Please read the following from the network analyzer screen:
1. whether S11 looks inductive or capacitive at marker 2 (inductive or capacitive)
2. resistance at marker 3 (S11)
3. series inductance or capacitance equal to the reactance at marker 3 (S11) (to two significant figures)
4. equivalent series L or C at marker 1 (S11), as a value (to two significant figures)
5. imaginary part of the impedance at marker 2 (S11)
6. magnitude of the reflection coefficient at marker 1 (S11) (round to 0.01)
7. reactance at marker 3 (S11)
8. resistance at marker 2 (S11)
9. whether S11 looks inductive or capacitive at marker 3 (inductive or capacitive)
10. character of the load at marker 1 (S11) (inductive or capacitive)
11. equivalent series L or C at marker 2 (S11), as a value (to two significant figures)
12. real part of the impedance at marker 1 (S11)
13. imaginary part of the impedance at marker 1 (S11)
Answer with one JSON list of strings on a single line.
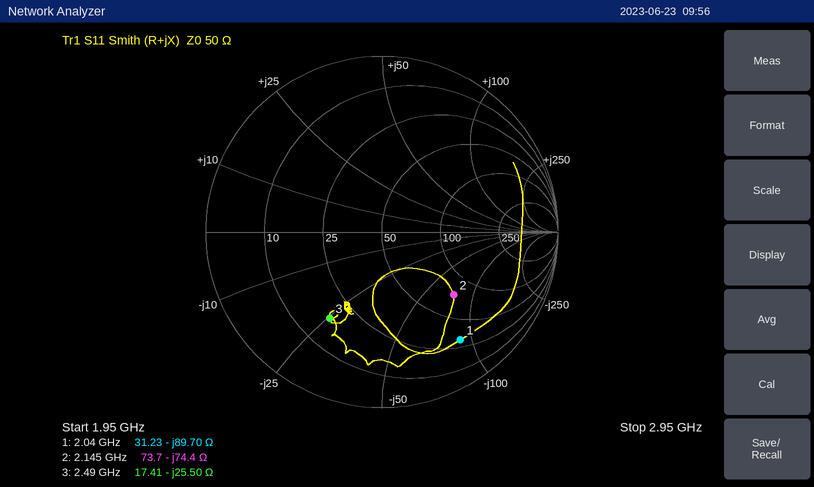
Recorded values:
["capacitive", "17.41 Ω", "2.5 pF", "870 fF", "-74.4 Ω", "0.76", "-25.50 Ω", "73.7 Ω", "capacitive", "capacitive", "1.00 pF", "31.23 Ω", "-89.70 Ω"]
